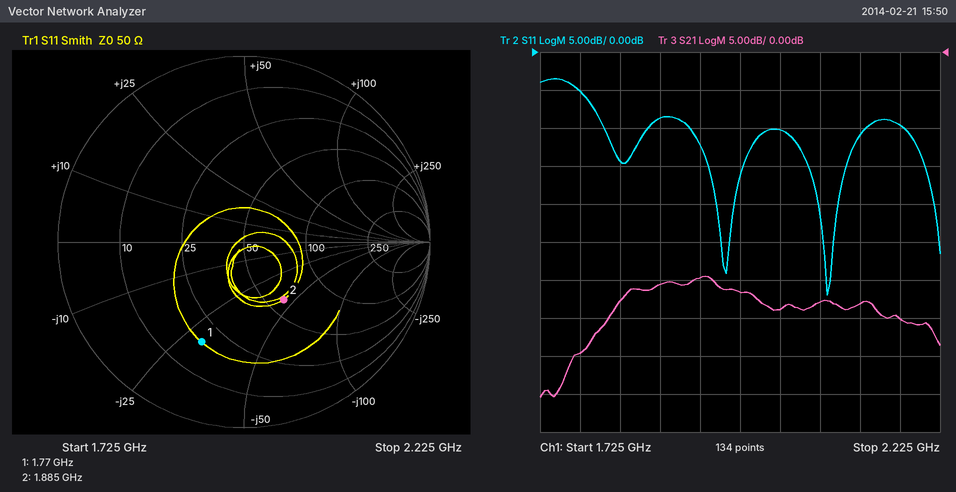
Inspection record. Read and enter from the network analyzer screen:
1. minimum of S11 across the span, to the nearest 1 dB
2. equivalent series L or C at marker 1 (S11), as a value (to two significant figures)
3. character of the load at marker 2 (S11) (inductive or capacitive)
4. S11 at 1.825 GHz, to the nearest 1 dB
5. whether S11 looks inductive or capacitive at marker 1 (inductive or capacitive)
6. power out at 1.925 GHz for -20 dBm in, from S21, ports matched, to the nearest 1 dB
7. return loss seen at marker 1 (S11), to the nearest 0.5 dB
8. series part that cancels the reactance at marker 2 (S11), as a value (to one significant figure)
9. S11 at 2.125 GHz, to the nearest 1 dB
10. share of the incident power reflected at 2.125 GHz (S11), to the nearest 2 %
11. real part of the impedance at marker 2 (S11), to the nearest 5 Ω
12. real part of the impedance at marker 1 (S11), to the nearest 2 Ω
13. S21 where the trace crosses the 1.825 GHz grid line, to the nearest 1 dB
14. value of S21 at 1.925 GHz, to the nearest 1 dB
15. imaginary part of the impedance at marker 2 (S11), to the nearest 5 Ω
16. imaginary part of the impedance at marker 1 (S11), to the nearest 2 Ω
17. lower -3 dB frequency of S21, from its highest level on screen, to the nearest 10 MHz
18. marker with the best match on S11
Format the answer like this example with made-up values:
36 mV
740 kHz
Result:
-32 dB
3.0 pF
capacitive
-14 dB
capacitive
-50 dBm
4.5 dB
4 nH
-11 dB
8 %
60 Ω
18 Ω
-33 dB
-30 dB
-45 Ω
-30 Ω
1.83 GHz
marker 2
